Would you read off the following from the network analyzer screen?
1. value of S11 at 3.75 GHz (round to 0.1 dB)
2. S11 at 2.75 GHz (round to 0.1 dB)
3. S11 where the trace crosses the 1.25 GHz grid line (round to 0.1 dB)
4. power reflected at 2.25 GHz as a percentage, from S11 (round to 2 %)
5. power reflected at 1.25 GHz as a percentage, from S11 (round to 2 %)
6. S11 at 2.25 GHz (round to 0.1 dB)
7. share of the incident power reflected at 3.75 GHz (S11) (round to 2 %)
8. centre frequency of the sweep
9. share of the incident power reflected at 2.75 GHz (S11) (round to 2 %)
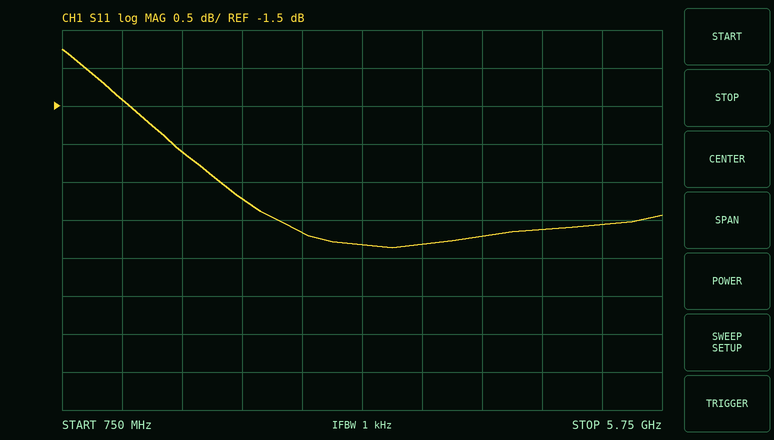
-3.3 dB
-3.2 dB
-1.4 dB
54 %
72 %
-2.7 dB
46 %
3.25 GHz
48 %
